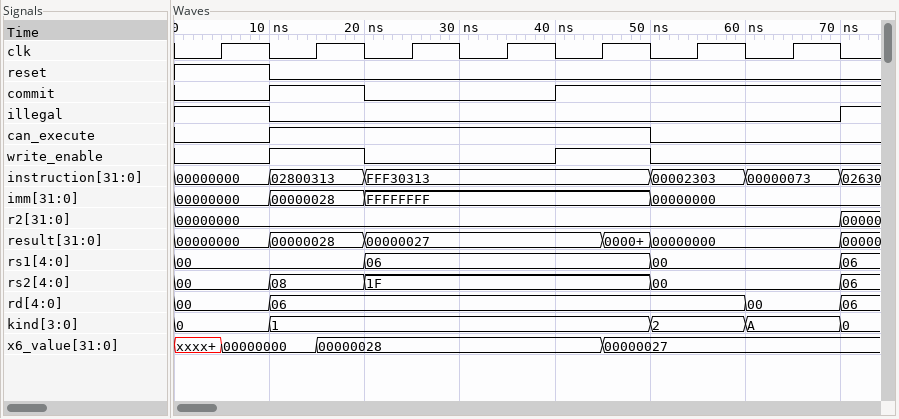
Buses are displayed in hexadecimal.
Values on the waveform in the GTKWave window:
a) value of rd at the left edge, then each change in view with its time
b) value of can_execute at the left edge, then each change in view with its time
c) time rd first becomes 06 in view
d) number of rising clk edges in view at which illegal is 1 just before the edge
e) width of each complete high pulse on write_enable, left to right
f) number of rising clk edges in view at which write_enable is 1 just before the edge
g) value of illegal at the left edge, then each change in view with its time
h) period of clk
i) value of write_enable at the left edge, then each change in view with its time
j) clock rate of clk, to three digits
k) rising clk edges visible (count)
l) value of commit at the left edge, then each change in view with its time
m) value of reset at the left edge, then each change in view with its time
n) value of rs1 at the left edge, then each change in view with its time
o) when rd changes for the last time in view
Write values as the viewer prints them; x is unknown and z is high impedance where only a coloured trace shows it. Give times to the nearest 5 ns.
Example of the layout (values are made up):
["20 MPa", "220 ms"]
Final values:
["00, 06 at 10 ns, 00 at 60 ns, 06 at 70 ns", "0, 1 at 10 ns, 0 at 50 ns", "10 ns", "1", "10 ns, 10 ns", "2", "1, 0 at 10 ns, 1 at 70 ns", "10 ns", "0, 1 at 10 ns, 0 at 20 ns, 1 at 40 ns, 0 at 50 ns", "100 MHz", "7", "0, 1 at 10 ns, 0 at 20 ns, 1 at 40 ns", "1, 0 at 10 ns", "00, 06 at 20 ns, 00 at 50 ns, 06 at 70 ns", "70 ns"]
